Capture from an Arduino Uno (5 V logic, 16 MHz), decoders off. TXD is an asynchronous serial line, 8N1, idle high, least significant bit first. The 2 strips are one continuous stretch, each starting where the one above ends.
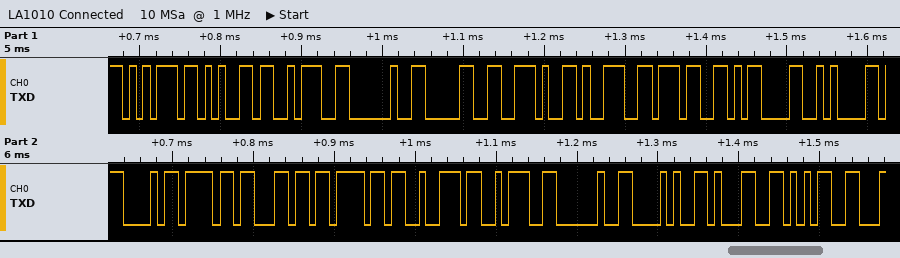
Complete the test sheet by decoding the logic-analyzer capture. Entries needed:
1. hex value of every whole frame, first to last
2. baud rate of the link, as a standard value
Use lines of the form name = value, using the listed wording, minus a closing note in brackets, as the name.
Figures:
hex value of every whole frame, first to last = 0x75 0x65 0x3A 0x20 0x30 0x2E 0x39 0x37 0x0D 0x0A 0x43 0x6F 0x6C 0x6F 0x72 0x3A 0x20 0x28 0x31 0x35
baud rate of the link, as a standard value = 115200 baud
